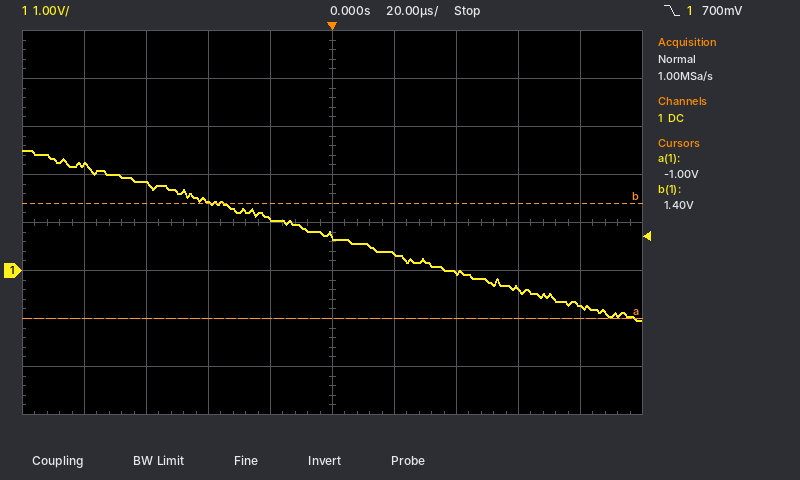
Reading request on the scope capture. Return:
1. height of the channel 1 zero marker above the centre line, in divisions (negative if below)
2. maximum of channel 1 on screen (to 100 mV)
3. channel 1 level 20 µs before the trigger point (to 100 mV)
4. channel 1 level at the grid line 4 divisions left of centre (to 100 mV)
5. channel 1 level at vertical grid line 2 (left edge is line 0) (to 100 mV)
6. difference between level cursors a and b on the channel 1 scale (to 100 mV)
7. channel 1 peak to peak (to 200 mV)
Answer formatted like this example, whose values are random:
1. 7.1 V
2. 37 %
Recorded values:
1. -1.0 div
2. 2.5 V
3. 1.1 V
4. 2.2 V
5. 1.8 V
6. 2.4 V
7. 3.6 V
